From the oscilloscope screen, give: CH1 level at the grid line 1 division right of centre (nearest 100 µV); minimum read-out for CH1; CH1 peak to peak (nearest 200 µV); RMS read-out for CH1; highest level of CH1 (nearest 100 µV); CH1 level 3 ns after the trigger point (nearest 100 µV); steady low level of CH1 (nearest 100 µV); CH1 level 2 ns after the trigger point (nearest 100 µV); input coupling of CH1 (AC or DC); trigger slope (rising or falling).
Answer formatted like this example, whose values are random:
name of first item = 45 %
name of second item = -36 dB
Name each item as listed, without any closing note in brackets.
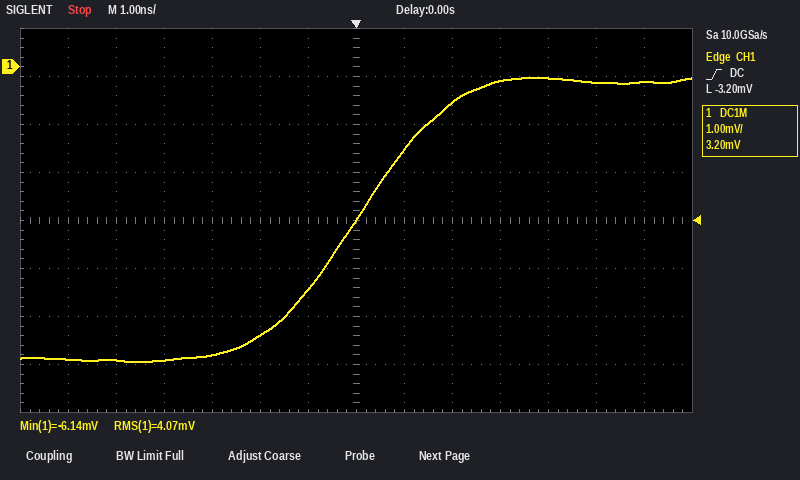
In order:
CH1 level at the grid line 1 division right of centre = -1.7 mV
minimum read-out for CH1 = -6.14 mV
CH1 peak to peak = 6.0 mV
RMS read-out for CH1 = 4.07 mV
highest level of CH1 = -200 µV
CH1 level 3 ns after the trigger point = -300 µV
steady low level of CH1 = -6.1 mV
CH1 level 2 ns after the trigger point = -700 µV
input coupling of CH1 = DC
trigger slope = rising
